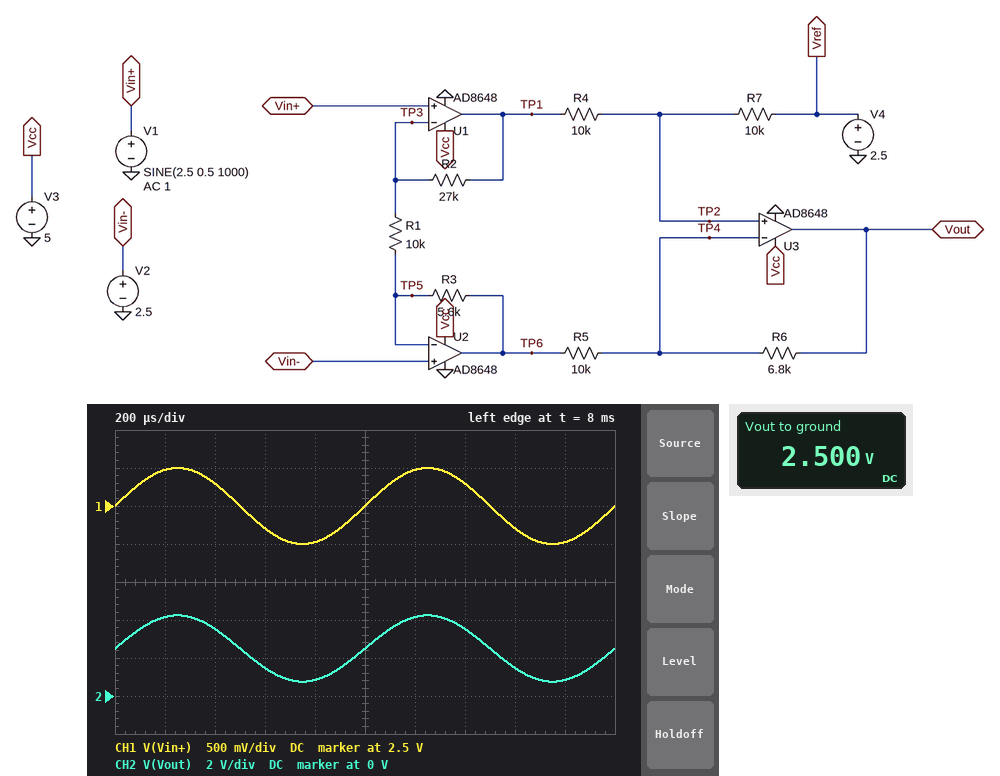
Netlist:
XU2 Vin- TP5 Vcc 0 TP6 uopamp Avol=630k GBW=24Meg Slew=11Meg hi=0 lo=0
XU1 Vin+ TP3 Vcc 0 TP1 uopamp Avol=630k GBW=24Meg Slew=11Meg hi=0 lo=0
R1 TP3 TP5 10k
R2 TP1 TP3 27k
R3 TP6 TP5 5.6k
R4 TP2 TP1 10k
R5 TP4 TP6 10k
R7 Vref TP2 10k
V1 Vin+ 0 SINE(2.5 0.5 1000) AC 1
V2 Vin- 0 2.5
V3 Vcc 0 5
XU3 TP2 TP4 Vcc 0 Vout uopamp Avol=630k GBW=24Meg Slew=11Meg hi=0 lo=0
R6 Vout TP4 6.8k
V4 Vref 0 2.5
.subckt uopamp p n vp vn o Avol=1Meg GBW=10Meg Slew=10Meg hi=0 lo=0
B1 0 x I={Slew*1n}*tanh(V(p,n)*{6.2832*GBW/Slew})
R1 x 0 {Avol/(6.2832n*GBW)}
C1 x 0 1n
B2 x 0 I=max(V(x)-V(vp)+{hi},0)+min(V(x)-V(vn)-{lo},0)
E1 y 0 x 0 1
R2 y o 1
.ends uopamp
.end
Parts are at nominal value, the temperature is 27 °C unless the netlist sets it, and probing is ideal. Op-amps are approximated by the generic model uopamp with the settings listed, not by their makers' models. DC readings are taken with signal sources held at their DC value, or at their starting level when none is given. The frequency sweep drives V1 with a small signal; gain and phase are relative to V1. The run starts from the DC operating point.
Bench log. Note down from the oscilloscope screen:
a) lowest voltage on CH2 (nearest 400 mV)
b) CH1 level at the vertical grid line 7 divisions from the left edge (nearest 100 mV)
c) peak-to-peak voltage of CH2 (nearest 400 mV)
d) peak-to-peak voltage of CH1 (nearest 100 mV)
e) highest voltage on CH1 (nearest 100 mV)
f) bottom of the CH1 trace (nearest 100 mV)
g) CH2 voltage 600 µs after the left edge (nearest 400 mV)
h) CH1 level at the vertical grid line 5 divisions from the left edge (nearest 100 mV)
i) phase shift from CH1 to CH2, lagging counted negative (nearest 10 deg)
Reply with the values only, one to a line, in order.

800 mV
2.8 V
3.6 V
1.0 V
3.0 V
2.0 V
1.6 V
2.5 V
0 deg
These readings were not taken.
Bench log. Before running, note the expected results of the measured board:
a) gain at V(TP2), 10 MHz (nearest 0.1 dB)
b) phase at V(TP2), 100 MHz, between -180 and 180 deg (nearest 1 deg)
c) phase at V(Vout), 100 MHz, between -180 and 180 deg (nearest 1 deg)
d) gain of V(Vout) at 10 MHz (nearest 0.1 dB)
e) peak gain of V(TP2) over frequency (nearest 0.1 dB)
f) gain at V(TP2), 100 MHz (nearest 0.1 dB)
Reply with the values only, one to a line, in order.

-0.6 dB
-85 deg
-168 deg
3.0 dB
5.3 dB
-18.5 dB
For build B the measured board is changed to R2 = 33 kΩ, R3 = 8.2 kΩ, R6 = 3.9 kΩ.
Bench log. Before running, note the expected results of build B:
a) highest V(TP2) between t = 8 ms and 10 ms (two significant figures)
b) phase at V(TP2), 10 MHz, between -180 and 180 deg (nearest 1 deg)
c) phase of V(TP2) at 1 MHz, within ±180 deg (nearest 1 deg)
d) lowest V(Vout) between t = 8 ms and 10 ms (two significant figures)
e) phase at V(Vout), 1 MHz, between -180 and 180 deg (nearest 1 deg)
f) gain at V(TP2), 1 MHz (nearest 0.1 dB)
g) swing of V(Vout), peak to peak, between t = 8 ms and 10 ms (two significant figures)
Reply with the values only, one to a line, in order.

3.6 V
-61 deg
-12 deg
850 mV
-15 deg
6.5 dB
3.3 V
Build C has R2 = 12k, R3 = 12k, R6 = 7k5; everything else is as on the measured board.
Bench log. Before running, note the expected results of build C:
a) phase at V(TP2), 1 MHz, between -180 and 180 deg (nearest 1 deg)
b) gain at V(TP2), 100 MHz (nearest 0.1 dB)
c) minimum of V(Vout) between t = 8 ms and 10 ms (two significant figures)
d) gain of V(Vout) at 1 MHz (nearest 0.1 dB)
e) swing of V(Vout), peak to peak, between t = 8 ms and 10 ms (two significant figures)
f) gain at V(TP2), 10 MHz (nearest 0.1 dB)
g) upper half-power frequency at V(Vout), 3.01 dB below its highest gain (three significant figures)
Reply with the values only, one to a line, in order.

-7 deg
-18.6 dB
1.1 V
8.9 dB
2.8 V
-3.1 dB
5.90 MHz
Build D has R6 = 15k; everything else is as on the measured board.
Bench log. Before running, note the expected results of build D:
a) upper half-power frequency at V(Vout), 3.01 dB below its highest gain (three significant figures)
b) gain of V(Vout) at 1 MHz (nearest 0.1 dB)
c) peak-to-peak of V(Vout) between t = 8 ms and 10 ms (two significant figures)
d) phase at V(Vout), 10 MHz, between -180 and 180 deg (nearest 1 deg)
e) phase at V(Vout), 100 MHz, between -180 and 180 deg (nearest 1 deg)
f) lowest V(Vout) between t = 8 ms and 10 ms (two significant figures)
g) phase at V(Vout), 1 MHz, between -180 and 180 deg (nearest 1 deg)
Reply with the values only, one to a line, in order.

4.50 MHz
14.6 dB
5.0 V
-107 deg
-172 deg
-9.1 mV
-16 deg
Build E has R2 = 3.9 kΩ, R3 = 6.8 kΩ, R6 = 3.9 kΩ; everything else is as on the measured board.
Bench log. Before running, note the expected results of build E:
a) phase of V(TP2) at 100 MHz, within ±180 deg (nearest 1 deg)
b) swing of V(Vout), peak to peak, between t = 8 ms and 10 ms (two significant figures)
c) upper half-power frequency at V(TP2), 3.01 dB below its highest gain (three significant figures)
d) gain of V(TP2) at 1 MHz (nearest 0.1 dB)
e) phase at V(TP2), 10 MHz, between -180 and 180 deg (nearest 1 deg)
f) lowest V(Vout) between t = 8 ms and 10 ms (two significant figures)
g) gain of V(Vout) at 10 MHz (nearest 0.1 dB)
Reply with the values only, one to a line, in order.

-79 deg
1.2 V
15.1 MHz
-3.2 dB
-32 deg
1.9 V
-1.6 dB
